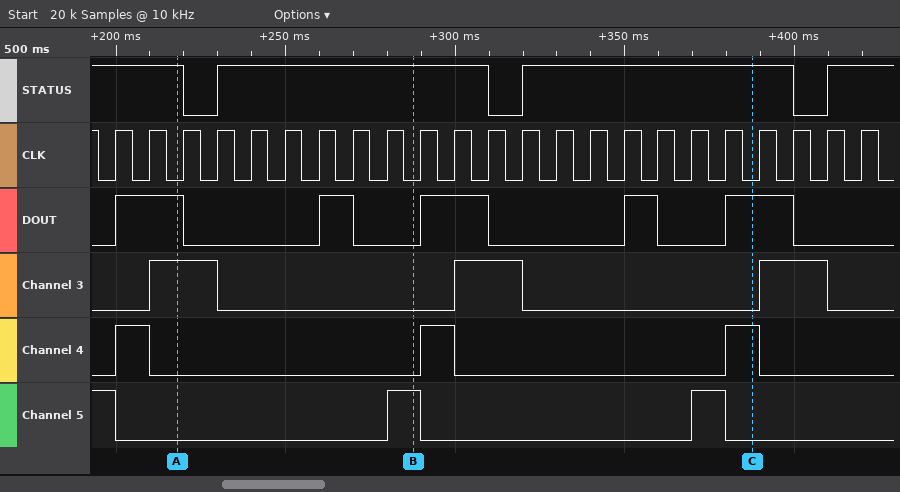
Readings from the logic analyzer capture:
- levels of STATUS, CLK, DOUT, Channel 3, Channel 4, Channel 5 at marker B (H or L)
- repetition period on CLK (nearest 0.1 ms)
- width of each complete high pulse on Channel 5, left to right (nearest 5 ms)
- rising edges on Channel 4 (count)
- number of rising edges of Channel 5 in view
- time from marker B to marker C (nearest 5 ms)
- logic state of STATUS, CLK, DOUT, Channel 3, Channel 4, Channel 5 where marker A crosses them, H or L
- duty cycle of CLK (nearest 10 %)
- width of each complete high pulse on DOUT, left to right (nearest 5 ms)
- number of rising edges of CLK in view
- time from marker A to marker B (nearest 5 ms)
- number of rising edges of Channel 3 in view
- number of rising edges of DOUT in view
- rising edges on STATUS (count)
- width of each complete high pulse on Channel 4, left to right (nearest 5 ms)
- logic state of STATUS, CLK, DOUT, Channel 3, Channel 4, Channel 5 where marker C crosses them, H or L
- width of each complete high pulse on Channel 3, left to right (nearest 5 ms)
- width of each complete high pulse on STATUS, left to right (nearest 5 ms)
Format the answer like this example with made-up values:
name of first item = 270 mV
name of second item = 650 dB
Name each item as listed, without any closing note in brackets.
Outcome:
levels of STATUS, CLK, DOUT, Channel 3, Channel 4, Channel 5 at marker B = STATUS=H, CLK=L, DOUT=L, Channel 3=L, Channel 4=L, Channel 5=H
repetition period on CLK = 10 ms
width of each complete high pulse on Channel 5, left to right = 10 ms, 10 ms
rising edges on Channel 4 = 3
number of rising edges of Channel 5 in view = 2
time from marker B to marker C = 100 ms
logic state of STATUS, CLK, DOUT, Channel 3, Channel 4, Channel 5 where marker A crosses them, H or L = STATUS=H, CLK=L, DOUT=H, Channel 3=H, Channel 4=L, Channel 5=L
duty cycle of CLK = 50 %
width of each complete high pulse on DOUT, left to right = 20 ms, 10 ms, 20 ms, 10 ms, 20 ms
number of rising edges of CLK in view = 23
time from marker A to marker B = 70 ms
number of rising edges of Channel 3 in view = 3
number of rising edges of DOUT in view = 5
rising edges on STATUS = 3
width of each complete high pulse on Channel 4, left to right = 10 ms, 10 ms, 10 ms
logic state of STATUS, CLK, DOUT, Channel 3, Channel 4, Channel 5 where marker C crosses them, H or L = STATUS=H, CLK=L, DOUT=H, Channel 3=L, Channel 4=H, Channel 5=L
width of each complete high pulse on Channel 3, left to right = 20 ms, 20 ms, 20 ms
width of each complete high pulse on STATUS, left to right = 80 ms, 80 ms
